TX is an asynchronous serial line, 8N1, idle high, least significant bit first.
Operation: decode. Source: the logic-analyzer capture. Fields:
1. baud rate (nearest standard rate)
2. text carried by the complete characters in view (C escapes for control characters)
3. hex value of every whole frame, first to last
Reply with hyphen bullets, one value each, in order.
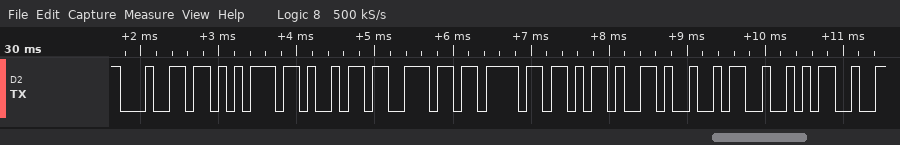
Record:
- 9600 baud
- "duino-IR"
- 0x64 0x75 0x69 0x6E 0x6F 0x2D 0x49 0x52
